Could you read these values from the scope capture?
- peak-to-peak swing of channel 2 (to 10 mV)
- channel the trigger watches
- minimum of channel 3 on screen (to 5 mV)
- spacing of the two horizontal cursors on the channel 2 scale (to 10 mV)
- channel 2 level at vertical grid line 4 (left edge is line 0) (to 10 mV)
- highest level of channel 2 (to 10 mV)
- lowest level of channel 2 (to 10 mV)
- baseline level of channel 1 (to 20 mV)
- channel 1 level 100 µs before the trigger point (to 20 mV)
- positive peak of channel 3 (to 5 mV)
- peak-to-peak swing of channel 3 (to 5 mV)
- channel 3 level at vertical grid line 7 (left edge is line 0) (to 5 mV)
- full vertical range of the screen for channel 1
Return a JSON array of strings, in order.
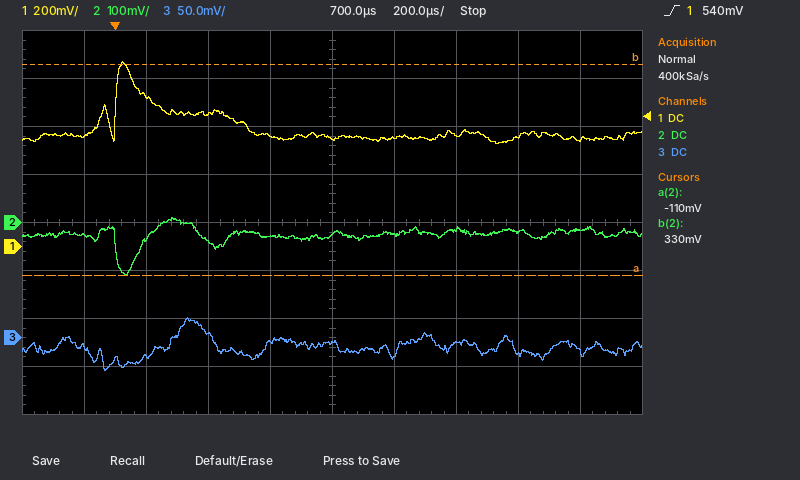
["120 mV", "channel 1", "-35 mV", "440 mV", "-30 mV", "10 mV", "-110 mV", "460 mV", "460 mV", "20 mV", "55 mV", "-5 mV", "1.6 V"]
